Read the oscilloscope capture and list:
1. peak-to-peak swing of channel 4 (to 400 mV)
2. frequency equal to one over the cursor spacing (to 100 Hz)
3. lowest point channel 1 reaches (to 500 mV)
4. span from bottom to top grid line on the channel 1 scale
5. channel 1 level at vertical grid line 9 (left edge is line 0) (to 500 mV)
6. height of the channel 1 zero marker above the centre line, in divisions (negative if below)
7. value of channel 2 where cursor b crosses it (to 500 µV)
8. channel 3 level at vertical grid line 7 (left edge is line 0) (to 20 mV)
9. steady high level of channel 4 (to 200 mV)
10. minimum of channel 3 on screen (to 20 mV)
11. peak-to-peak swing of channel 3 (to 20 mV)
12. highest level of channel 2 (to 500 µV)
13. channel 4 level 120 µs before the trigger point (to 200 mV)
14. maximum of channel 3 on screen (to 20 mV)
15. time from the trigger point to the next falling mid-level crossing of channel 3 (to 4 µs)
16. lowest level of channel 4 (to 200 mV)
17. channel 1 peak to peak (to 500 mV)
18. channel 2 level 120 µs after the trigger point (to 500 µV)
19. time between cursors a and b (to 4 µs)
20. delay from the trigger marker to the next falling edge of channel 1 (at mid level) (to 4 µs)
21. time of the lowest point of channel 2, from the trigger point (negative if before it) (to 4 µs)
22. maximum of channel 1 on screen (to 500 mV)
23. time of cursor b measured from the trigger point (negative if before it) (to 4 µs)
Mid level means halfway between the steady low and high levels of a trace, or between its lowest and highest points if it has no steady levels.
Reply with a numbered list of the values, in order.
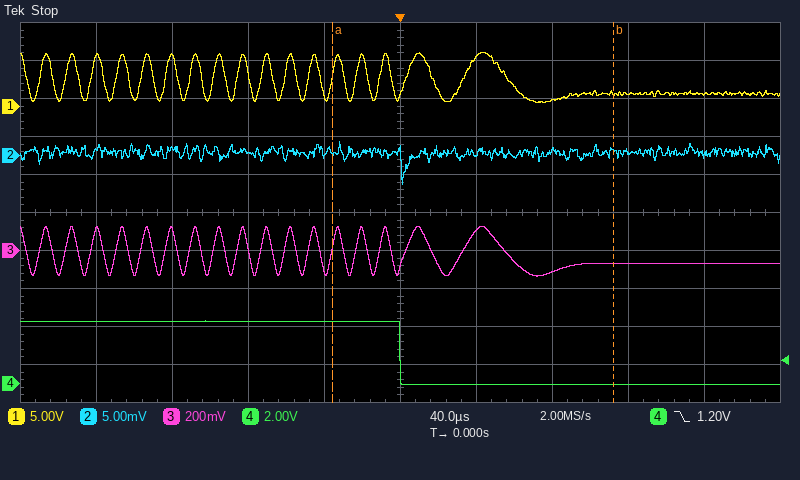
1. 3.2 V
2. 6.8 kHz
3. 500 mV
4. 50 V
5. 1.5 V
6. +2.8 div
7. 500 µV
8. -120 mV
9. 3.2 V
10. -140 mV
11. 260 mV
12. 2.0 mV
13. 3.2 V
14. 120 mV
15. 16 µs
16. 0.0 V
17. 6.5 V
18. 500 µV
19. 148 µs
20. 16 µs
21. 0 µs
22. 7.0 V
23. +112 µs
